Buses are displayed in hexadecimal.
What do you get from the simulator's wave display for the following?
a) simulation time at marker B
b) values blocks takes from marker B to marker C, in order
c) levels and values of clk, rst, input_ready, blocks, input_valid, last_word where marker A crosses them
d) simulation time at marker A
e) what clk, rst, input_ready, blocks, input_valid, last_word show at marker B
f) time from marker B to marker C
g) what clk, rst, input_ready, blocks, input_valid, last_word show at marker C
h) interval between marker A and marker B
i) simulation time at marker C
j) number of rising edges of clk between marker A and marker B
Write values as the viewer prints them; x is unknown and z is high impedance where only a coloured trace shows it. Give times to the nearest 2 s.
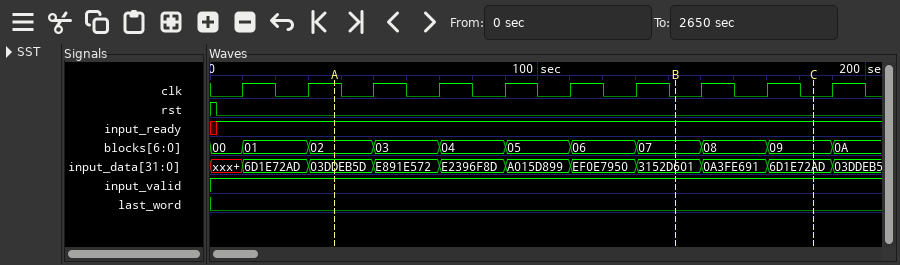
142 s
07, 08, 09
clk=1, rst=0, input_ready=1, blocks=02, input_valid=1, last_word=0
38 s
clk=0, rst=0, input_ready=1, blocks=07, input_valid=1, last_word=0
42 s
clk=0, rst=0, input_ready=1, blocks=09, input_valid=1, last_word=0
104 s
184 s
5
